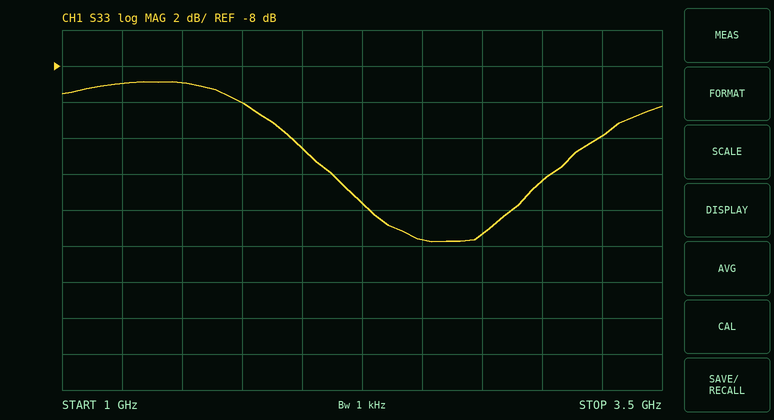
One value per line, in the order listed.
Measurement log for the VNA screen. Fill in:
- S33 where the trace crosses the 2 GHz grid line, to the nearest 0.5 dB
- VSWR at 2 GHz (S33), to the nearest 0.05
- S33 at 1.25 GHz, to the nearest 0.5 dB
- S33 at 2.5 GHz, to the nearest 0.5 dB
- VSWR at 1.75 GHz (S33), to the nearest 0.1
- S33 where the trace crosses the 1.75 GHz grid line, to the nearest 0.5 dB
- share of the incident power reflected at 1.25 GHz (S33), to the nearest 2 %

-12.5 dB
1.60
-9.0 dB
-17.5 dB
1.9
-10.0 dB
12 %
